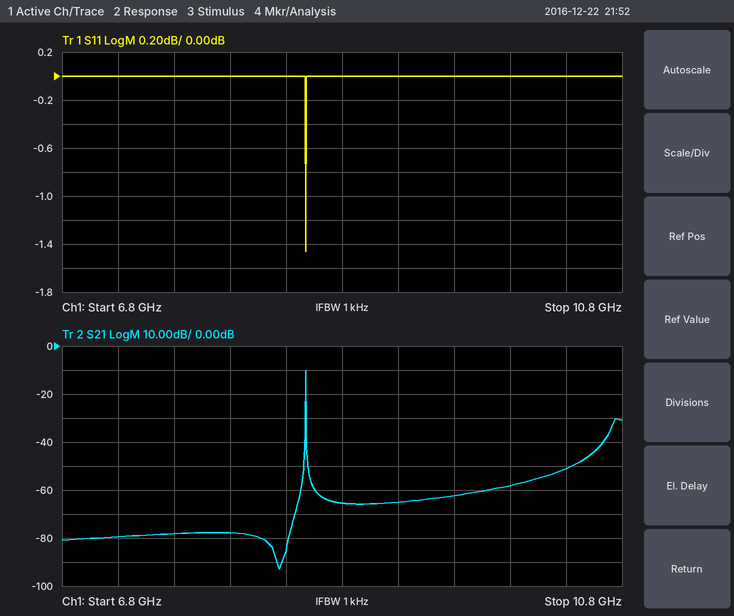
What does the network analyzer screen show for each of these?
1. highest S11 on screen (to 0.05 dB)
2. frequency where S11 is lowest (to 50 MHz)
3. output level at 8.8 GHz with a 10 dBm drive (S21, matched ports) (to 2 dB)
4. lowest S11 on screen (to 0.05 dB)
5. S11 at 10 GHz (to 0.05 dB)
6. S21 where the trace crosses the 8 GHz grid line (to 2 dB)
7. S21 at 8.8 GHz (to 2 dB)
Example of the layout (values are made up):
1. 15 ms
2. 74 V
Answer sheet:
1. 0.00 dB
2. 8.55 GHz
3. -56 dBm
4. -1.45 dB
5. 0.00 dB
6. -78 dB
7. -66 dB
